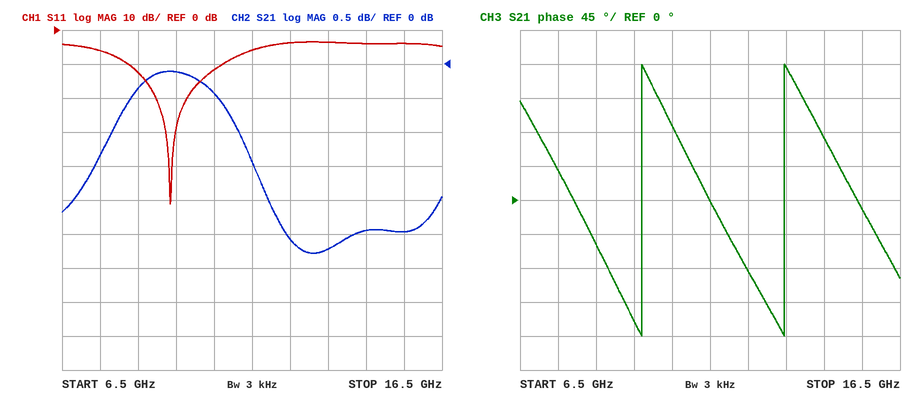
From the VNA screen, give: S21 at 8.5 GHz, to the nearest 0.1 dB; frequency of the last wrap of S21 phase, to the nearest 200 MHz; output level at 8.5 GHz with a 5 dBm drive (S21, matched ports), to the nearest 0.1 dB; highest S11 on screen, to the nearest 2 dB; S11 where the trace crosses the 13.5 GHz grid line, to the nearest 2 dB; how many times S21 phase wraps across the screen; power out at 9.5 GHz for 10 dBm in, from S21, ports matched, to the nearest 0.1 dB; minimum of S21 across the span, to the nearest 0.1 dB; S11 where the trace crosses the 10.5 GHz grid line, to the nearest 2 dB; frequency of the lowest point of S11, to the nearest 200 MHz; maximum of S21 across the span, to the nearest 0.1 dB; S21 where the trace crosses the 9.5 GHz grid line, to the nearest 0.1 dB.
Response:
-0.4 dB
13.4 GHz
4.6 dBm
-4 dB
-4 dB
2
9.9 dBm
-2.8 dB
-12 dB
9.4 GHz
-0.1 dB
-0.1 dB
